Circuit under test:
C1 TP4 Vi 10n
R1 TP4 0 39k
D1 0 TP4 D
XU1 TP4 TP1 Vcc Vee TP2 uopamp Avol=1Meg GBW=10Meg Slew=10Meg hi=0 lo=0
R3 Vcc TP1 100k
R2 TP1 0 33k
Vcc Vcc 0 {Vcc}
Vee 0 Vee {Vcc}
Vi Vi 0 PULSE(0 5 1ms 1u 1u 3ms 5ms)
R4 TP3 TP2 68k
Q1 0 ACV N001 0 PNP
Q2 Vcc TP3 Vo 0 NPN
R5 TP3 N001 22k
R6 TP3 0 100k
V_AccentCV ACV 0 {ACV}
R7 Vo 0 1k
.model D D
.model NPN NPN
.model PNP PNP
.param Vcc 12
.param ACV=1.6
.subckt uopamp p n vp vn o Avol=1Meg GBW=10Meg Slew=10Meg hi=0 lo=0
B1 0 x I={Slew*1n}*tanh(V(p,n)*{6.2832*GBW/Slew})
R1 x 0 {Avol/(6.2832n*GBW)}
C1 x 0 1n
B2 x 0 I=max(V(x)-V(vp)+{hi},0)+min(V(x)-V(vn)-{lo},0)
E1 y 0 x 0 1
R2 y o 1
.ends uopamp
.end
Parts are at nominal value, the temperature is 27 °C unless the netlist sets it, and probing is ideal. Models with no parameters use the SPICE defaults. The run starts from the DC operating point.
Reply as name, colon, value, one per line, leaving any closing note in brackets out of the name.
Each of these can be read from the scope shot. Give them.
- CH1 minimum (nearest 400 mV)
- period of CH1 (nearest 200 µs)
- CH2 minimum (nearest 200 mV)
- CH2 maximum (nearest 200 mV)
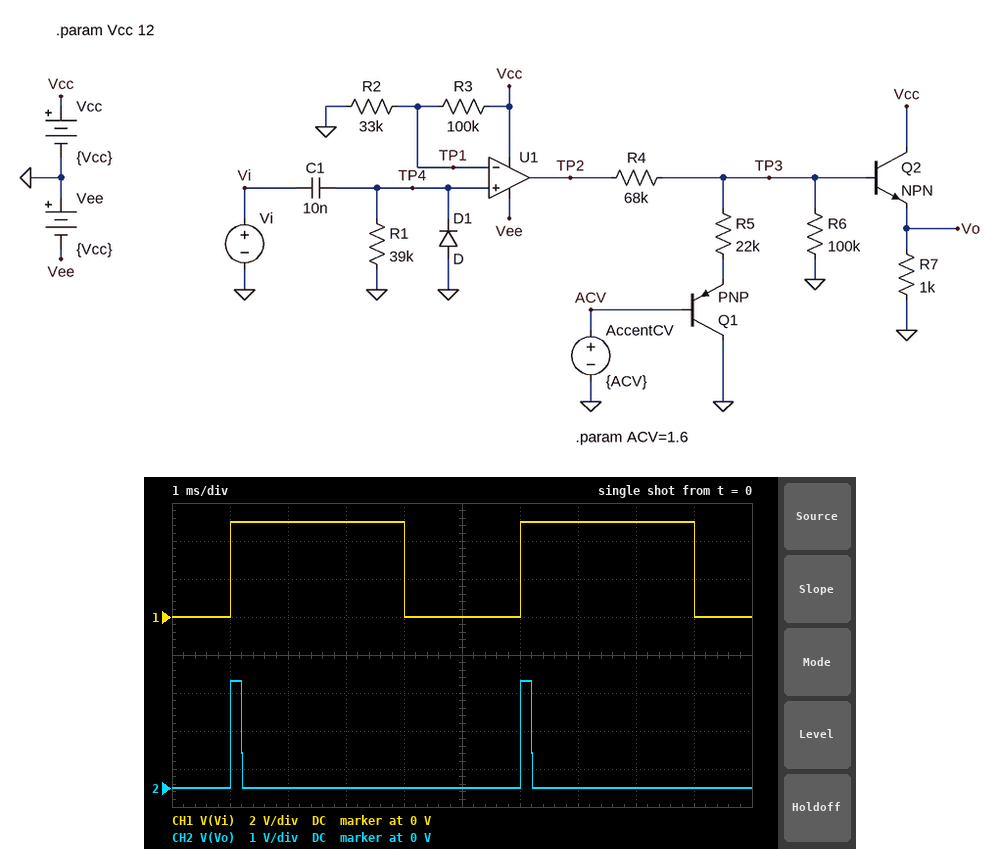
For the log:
CH1 minimum: 0 V
period of CH1: 5.0 ms
CH2 minimum: 0 V
CH2 maximum: 2.8 V
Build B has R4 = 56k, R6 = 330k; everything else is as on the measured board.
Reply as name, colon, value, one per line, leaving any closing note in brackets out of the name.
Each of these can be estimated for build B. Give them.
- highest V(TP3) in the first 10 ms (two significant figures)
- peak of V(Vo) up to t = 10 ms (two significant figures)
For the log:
highest V(TP3) in the first 10 ms: 4.3 V
peak of V(Vo) up to t = 10 ms: 3.5 V
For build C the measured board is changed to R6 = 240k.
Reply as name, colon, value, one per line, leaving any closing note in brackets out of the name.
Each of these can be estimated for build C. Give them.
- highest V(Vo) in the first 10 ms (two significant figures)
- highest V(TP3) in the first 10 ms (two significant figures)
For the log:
highest V(Vo) in the first 10 ms: 3.1 V
highest V(TP3) in the first 10 ms: 3.9 V
